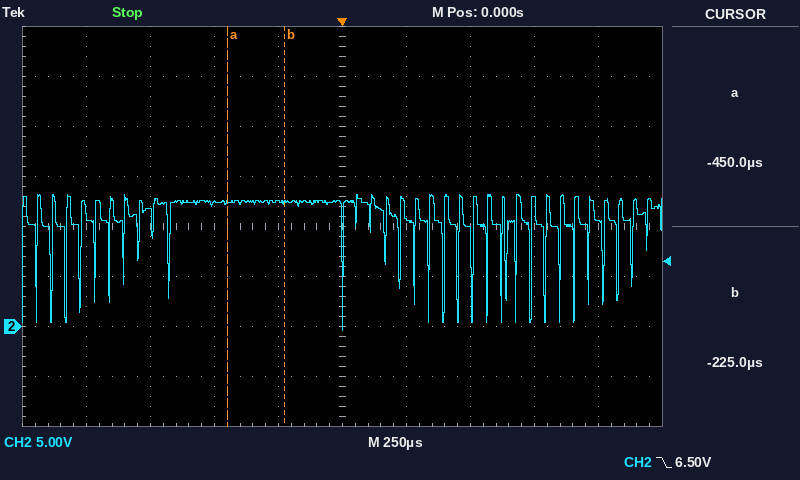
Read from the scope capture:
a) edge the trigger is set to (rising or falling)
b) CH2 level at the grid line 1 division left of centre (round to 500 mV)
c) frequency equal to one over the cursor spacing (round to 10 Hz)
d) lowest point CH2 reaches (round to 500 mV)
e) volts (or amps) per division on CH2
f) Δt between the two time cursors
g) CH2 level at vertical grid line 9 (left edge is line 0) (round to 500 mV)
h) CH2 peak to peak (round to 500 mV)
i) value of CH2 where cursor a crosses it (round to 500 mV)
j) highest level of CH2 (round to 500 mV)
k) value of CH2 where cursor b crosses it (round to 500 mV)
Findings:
falling
12.5 V
4.44 kHz
-500 mV
5 V
225 µs
10.5 V
13.5 V
12.5 V
13.0 V
12.5 V
